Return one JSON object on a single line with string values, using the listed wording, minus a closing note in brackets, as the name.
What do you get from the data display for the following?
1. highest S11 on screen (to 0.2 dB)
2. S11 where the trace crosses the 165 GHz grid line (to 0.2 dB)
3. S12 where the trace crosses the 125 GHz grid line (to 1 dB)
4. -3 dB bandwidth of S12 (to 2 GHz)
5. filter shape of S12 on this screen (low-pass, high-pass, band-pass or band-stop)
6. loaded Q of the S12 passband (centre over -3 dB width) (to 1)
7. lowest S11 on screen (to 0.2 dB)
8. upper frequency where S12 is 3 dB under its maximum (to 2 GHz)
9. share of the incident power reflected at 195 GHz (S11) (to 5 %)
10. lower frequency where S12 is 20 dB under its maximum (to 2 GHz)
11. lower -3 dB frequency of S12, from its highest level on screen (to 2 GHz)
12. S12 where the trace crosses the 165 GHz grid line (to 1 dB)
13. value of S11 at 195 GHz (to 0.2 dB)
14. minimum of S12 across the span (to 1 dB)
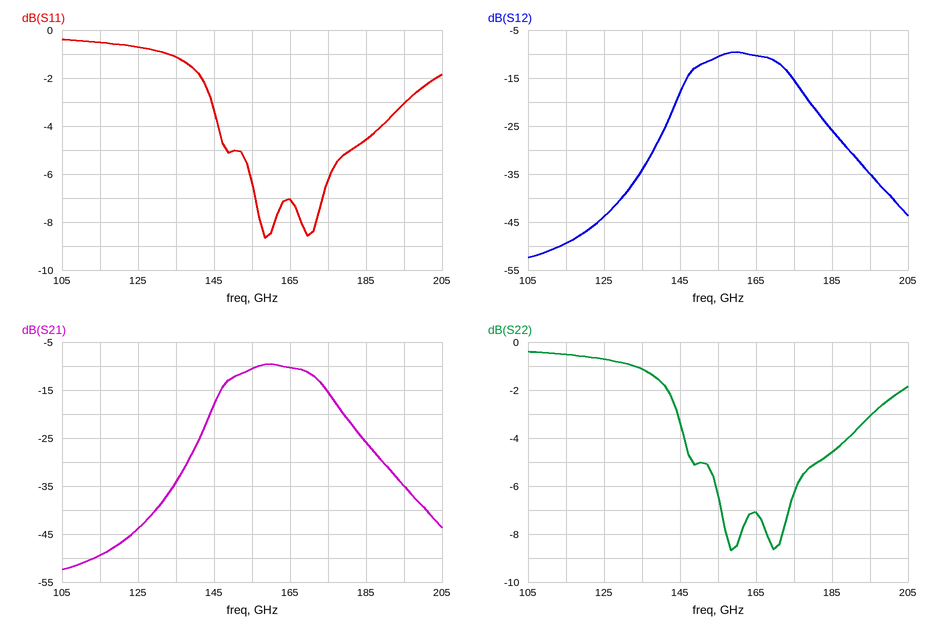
{"highest S11 on screen": "-0.4 dB", "S11 where the trace crosses the 165 GHz grid line": "-7.0 dB", "S12 where the trace crosses the 125 GHz grid line": "-44 dB", "-3 dB bandwidth of S12": "22 GHz", "filter shape of S12 on this screen": "band-pass", "loaded Q of the S12 passband (centre over -3 dB width)": "7", "lowest S11 on screen": "-8.6 dB", "upper frequency where S12 is 3 dB under its maximum": "172 GHz", "share of the incident power reflected at 195 GHz (S11)": "50 %", "lower frequency where S12 is 20 dB under its maximum": "138 GHz", "lower -3 dB frequency of S12, from its highest level on screen": "150 GHz", "S12 where the trace crosses the 165 GHz grid line": "-10 dB", "value of S11 at 195 GHz": "-3.0 dB", "minimum of S12 across the span": "-52 dB"}
